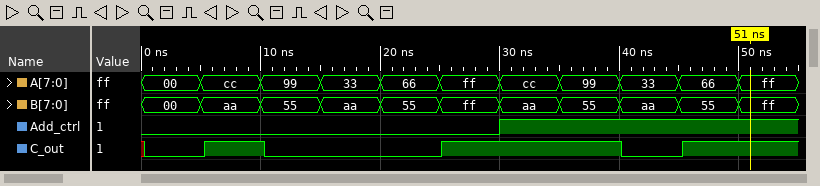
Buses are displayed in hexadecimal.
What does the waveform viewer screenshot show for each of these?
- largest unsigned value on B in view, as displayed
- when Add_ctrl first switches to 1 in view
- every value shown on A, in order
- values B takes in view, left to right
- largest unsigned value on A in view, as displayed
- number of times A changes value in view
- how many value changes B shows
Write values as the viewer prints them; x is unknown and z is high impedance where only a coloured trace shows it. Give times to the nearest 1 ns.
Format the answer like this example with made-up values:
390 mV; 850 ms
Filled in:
ff; 30 ns; 00, cc, 99, 33, 66, ff, cc, 99, 33, 66, ff; 00, aa, 55, aa, 55, ff, aa, 55, aa, 55, ff; ff; 10; 10
